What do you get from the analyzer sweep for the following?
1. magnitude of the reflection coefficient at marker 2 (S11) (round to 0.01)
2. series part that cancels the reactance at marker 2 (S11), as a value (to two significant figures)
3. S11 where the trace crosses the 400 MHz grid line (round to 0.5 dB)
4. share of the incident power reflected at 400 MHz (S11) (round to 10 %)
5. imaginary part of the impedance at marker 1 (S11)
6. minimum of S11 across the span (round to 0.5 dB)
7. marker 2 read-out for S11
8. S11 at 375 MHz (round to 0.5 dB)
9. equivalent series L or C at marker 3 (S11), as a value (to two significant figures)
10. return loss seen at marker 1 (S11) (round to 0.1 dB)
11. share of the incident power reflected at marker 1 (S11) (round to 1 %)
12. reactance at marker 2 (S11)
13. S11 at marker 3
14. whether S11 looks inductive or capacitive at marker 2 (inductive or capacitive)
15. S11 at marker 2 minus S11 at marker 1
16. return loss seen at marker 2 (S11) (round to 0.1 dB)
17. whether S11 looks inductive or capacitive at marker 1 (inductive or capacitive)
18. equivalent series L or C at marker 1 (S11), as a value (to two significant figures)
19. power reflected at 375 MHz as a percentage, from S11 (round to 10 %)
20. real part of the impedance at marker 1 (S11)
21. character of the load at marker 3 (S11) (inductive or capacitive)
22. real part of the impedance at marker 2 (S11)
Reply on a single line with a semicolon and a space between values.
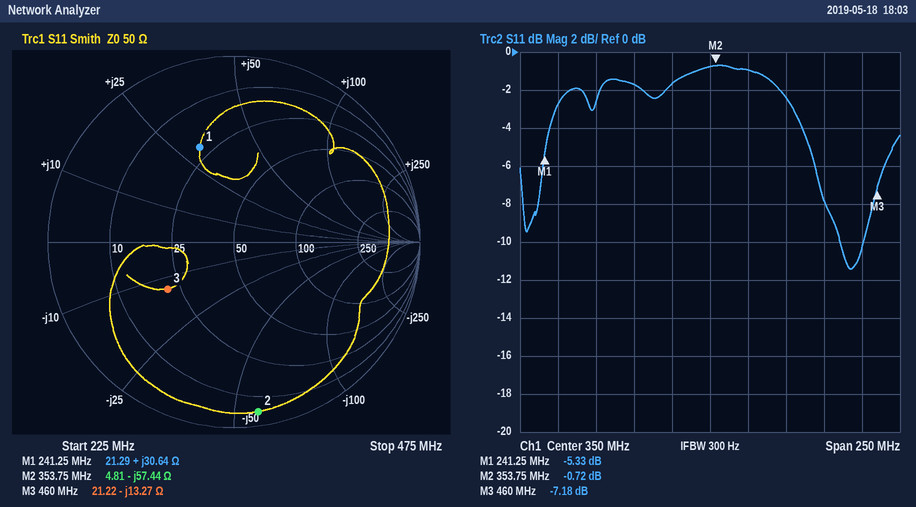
0.92; 26 nH; -2.5 dB; 60 %; +30.64 Ω; -11.5 dB; -0.72 dB; -1.0 dB; 26 pF; 5.3 dB; 29 %; -57.44 Ω; -7.18 dB; capacitive; 4.61 dB; 0.7 dB; inductive; 20 nH; 80 %; 21.29 Ω; capacitive; 4.81 Ω
